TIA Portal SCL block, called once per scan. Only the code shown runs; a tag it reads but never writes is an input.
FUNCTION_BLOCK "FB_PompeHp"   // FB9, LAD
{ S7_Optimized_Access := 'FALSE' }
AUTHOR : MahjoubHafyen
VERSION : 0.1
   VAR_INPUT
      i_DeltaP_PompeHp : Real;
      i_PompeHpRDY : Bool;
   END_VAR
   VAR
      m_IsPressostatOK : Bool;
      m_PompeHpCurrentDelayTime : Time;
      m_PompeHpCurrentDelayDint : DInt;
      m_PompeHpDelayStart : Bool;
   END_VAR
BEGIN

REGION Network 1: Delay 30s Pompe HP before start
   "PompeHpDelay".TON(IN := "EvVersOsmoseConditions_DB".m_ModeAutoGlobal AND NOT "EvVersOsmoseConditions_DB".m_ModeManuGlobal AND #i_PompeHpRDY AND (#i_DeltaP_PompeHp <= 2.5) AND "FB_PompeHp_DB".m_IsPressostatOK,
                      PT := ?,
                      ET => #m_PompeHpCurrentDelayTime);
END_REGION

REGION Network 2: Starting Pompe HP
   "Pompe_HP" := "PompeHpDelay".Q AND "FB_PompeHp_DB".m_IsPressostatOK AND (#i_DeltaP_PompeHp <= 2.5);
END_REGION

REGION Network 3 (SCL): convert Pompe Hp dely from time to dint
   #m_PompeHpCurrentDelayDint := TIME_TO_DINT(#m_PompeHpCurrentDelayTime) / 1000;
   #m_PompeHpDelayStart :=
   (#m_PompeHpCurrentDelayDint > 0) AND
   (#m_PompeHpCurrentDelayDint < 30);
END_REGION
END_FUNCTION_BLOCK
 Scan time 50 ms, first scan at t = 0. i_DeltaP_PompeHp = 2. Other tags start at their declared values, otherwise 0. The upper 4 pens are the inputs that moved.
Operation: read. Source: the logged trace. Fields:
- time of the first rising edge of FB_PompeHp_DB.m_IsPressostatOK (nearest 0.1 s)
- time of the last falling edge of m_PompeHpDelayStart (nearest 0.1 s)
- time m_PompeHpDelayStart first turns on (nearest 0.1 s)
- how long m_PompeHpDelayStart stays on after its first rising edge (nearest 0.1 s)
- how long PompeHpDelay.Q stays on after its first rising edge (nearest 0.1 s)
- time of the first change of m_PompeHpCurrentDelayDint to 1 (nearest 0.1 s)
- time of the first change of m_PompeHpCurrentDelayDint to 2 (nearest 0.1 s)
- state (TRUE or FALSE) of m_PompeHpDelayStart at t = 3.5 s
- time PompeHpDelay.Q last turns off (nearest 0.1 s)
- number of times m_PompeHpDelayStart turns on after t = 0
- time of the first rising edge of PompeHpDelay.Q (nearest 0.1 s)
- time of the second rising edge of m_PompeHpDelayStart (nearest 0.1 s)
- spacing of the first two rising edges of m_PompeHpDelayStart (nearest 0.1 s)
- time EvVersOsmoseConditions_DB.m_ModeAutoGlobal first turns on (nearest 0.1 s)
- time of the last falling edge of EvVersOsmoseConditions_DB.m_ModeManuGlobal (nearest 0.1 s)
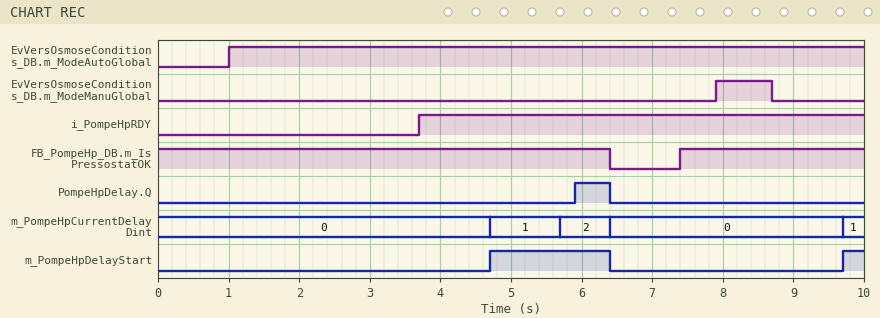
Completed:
7.4 s
6.4 s
4.7 s
1.7 s
0.5 s
4.7 s
5.7 s
FALSE
6.4 s
2
5.9 s
9.7 s
5.0 s
1.0 s
8.7 s
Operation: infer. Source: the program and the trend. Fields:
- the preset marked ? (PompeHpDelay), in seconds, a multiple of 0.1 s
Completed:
2.2 s
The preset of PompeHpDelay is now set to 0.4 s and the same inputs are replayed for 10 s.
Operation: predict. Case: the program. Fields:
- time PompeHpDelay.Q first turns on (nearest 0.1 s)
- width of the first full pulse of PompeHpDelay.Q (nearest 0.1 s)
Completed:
4.1 s
2.3 s
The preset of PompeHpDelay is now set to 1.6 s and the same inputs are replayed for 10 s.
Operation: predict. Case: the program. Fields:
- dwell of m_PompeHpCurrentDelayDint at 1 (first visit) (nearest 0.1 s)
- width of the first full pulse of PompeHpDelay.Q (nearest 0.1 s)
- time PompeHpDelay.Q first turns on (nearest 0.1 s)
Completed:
1.7 s
1.1 s
5.3 s
